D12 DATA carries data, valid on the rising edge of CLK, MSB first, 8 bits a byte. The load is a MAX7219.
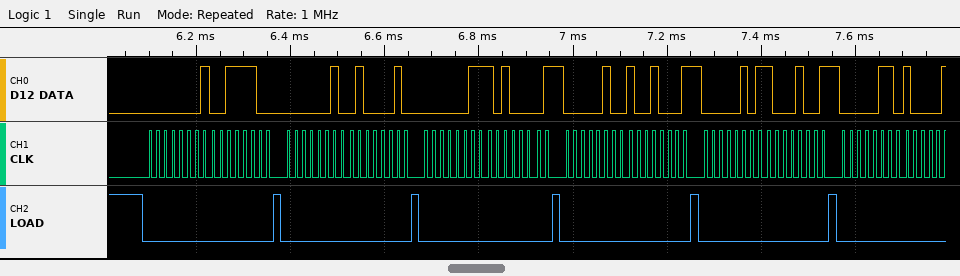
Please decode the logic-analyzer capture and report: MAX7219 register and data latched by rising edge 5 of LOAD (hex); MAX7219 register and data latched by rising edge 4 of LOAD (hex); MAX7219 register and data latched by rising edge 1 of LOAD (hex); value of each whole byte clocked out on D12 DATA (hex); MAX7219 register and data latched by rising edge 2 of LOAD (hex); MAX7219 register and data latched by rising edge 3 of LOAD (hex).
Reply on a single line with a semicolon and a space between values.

register 0x5, data 0x89; register 0x4, data 0x91; register 0x1, data 0x3C; 01 3C 02 42 03 A1 04 91 05 89 06; register 0x2, data 0x42; register 0x3, data 0xA1
